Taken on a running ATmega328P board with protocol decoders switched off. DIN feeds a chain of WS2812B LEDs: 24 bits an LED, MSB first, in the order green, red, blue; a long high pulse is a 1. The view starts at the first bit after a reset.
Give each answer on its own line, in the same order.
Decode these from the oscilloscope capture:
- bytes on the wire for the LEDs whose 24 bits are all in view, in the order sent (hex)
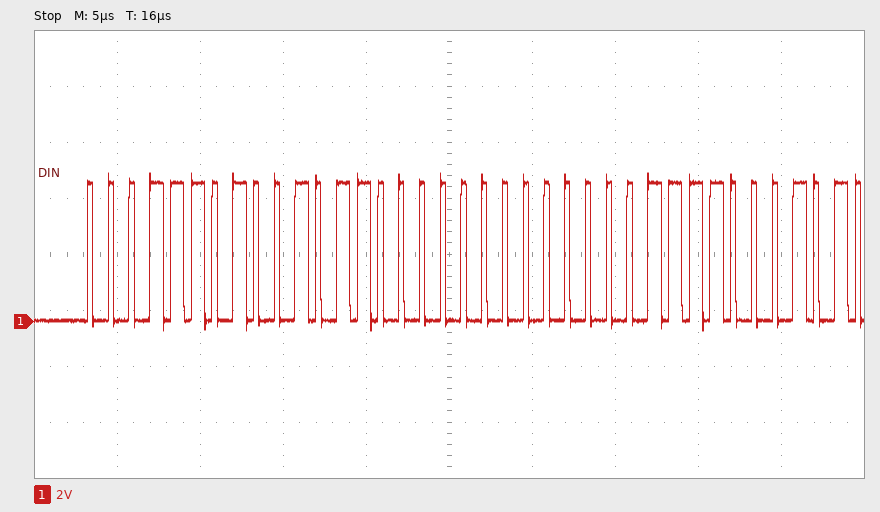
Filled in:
1D 2C 00
